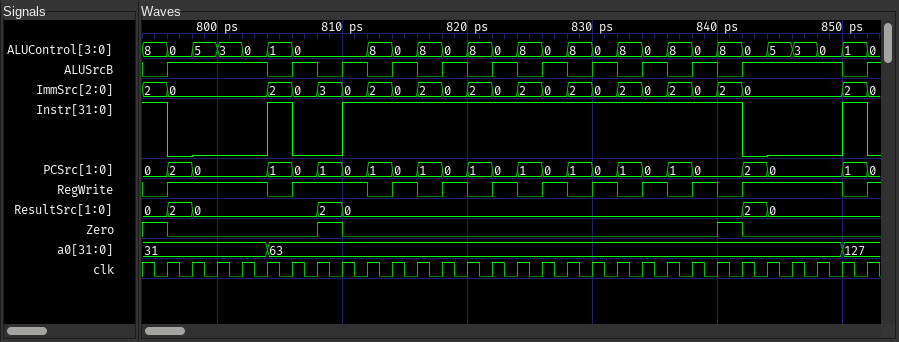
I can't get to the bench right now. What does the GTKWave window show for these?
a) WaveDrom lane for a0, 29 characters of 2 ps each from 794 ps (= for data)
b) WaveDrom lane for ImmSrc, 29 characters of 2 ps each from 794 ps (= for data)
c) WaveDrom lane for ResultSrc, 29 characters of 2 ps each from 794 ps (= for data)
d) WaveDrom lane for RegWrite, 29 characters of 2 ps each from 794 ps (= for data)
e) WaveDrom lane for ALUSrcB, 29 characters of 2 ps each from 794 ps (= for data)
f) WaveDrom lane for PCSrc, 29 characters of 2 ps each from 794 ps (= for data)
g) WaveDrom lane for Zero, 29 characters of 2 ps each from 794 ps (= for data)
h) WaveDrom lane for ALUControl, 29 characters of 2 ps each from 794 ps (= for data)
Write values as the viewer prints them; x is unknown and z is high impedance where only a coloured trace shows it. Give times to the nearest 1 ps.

{name: 'a0', wave: '=....=......................=', data: '31 63 127'}
{name: 'ImmSrc', wave: '==...====================...=', data: '2 0 2 0 3 0 2 0 2 0 2 0 2 0 2 0 2 0 2 0 2 0 2'}
{name: 'ResultSrc', wave: '===....==...............==...', data: '0 2 0 2 0 2 0'}
{name: 'RegWrite', wave: '01...01..0101010101010101...0'}
{name: 'ALUSrcB', wave: '01...01010101010101010101...0'}
{name: 'PCSrc', wave: '===..==================.==..=', data: '0 2 0 1 0 1 0 1 0 1 0 1 0 1 0 1 0 1 0 1 0 2 0 1'}
{name: 'Zero', wave: '10.....10..............10....'}
{name: 'ALUControl', wave: '=======..====================', data: '8 0 5 3 0 1 0 8 0 8 0 8 0 8 0 8 0 8 0 8 0 8 0 5 3 0 1'}
